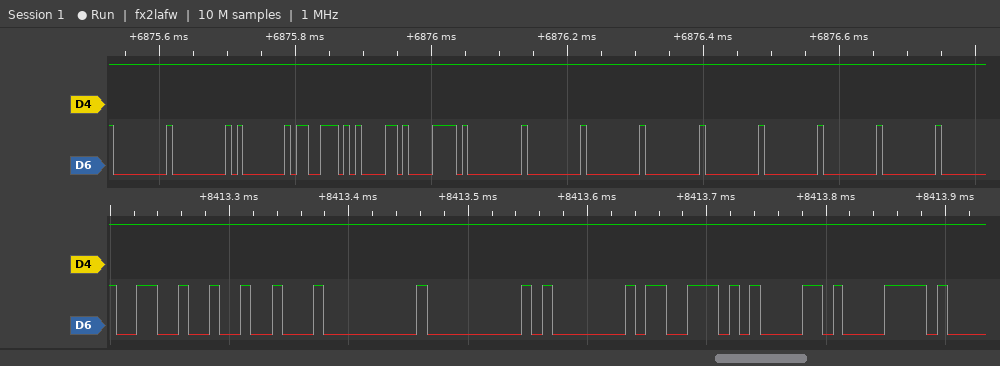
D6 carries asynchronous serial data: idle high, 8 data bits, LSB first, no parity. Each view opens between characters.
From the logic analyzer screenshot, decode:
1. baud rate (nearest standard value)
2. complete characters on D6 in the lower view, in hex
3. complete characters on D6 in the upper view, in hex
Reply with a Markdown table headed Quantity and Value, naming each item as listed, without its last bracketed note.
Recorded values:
| Quantity | Value |
|---|---|
| baud rate | 115200 baud |
| complete characters on D6 in the lower view, in hex | 26, 12, 00, 00, 01, 73, 61, 78 |
| complete characters on D6 in the upper view, in hex | 00, 00, 01, 73, 61, 78, 00, 00, 00, 00, 00, 00, 00, 00 |
